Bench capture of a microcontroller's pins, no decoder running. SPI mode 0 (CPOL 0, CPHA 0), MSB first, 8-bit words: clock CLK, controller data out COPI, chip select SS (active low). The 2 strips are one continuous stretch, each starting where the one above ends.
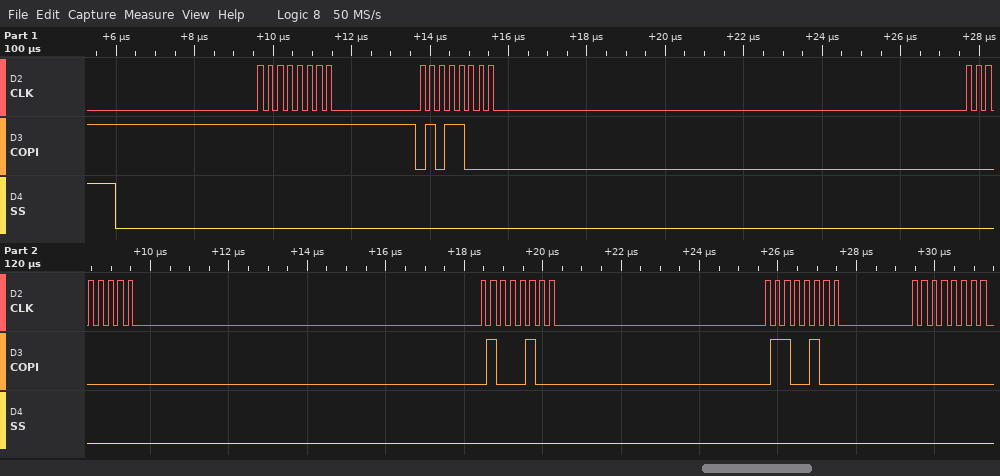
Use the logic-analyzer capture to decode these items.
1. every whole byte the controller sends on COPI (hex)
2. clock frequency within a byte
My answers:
FF 58 00 44 64 00
4 MHz
